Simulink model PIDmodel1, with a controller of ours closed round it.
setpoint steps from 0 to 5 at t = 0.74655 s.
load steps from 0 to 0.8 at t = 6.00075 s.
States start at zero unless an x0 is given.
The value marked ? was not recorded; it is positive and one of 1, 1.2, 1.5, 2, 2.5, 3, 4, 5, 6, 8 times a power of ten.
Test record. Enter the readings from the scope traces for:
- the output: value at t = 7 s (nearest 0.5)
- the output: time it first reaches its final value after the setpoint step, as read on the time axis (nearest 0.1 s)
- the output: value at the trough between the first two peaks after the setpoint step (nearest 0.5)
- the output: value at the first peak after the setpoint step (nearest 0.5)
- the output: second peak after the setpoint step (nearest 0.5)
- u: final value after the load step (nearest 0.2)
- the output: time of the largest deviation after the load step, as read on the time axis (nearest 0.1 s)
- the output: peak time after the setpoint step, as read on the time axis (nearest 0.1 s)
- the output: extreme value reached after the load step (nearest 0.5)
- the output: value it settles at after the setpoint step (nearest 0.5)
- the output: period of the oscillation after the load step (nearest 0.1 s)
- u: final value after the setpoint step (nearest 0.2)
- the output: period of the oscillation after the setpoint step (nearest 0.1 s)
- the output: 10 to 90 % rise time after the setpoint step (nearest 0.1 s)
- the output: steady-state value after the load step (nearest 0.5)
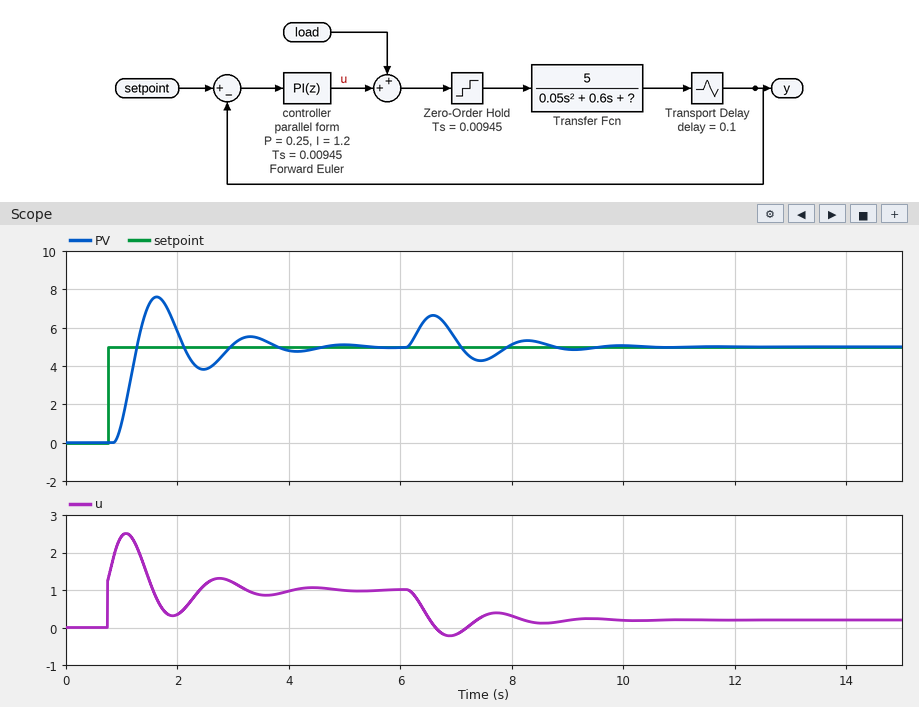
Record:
5.5
1.3 s
4.0
7.5
5.5
0.2
6.6 s
1.6 s
6.5
5.0
1.7 s
1.0
1.7 s
0.3 s
5.0
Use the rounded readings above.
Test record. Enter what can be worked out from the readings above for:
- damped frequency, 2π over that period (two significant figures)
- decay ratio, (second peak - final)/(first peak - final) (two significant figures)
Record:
3.7 rad/s
0.20
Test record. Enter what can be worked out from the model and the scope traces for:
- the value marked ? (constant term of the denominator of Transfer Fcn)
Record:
1
